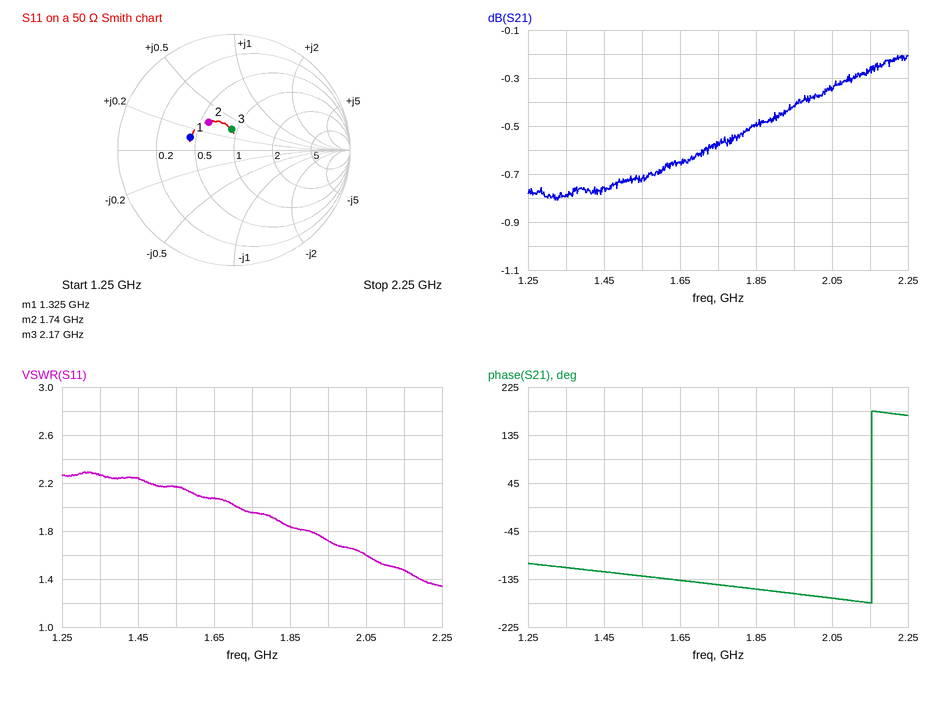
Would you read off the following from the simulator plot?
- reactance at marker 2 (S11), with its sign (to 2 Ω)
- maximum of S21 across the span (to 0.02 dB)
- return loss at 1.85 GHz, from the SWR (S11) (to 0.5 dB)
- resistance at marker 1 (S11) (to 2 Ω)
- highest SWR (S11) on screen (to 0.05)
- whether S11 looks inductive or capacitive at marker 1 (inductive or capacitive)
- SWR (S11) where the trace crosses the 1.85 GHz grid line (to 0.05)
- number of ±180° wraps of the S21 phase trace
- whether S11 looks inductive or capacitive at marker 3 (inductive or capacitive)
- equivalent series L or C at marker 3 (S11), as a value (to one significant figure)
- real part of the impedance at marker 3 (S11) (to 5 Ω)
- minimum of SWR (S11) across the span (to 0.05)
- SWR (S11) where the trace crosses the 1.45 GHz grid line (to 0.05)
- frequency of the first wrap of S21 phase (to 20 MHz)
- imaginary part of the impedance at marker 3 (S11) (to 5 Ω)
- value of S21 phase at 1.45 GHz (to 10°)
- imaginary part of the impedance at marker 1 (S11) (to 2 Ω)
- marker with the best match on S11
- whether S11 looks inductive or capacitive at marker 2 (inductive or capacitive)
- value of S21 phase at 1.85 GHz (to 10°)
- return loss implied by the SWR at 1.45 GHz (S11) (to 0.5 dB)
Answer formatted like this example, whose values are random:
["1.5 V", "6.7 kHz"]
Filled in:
["+16 Ω", "-0.20 dB", "10.5 dB", "22 Ω", "2.30", "inductive", "1.85", "1", "inductive", "1 nH", "45 Ω", "1.35", "2.25", "2.16 GHz", "+15 Ω", "-120°", "+6 Ω", "marker 3", "inductive", "-150°", "8.5 dB"]
